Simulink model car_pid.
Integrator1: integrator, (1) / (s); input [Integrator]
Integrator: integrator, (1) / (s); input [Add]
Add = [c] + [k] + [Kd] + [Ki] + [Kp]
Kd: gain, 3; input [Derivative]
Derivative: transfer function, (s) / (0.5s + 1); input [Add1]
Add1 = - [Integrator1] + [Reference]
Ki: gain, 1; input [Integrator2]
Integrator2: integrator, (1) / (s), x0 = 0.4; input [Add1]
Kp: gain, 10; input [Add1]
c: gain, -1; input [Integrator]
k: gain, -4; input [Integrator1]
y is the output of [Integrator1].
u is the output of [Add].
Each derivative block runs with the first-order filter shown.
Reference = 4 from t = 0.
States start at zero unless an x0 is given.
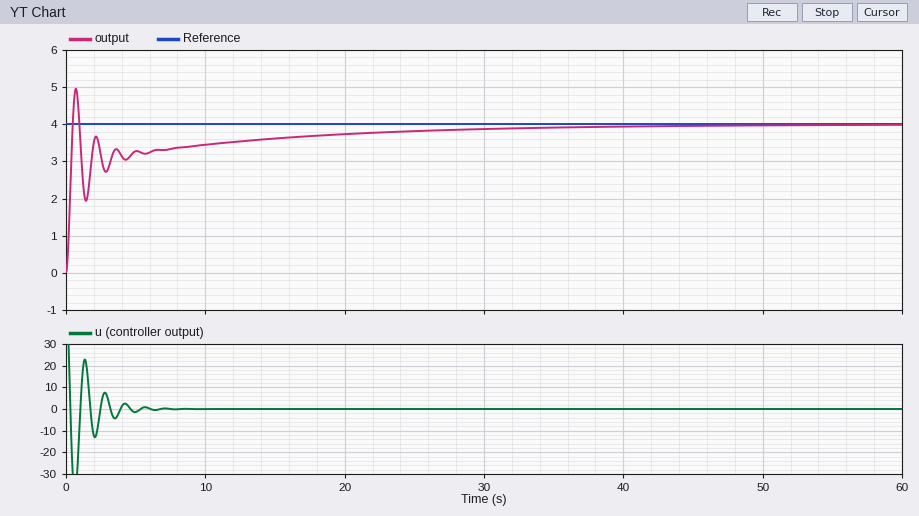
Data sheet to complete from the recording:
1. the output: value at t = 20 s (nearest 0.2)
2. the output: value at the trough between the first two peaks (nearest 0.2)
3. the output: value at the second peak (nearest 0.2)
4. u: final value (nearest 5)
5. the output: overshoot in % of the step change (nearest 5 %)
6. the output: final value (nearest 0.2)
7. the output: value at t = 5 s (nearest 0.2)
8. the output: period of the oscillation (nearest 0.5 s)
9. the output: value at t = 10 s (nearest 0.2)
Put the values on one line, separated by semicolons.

3.8; 2.0; 3.6; 0; 25 %; 4.0; 3.2; 1.5 s; 3.4
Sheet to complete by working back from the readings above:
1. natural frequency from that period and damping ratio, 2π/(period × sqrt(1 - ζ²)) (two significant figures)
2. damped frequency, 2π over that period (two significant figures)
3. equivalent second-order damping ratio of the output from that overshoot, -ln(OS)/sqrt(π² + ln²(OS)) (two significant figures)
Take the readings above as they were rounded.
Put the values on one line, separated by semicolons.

4.6 rad/s; 4.2 rad/s; 0.40
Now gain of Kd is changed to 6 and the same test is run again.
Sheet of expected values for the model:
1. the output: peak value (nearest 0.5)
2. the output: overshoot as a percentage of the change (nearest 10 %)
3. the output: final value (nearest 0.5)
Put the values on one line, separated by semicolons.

5.0; 30 %; 4.0
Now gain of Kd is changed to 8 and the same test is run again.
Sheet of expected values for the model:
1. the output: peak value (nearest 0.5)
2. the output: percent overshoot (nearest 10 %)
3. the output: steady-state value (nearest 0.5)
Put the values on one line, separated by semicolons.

5.0; 30 %; 4.0
